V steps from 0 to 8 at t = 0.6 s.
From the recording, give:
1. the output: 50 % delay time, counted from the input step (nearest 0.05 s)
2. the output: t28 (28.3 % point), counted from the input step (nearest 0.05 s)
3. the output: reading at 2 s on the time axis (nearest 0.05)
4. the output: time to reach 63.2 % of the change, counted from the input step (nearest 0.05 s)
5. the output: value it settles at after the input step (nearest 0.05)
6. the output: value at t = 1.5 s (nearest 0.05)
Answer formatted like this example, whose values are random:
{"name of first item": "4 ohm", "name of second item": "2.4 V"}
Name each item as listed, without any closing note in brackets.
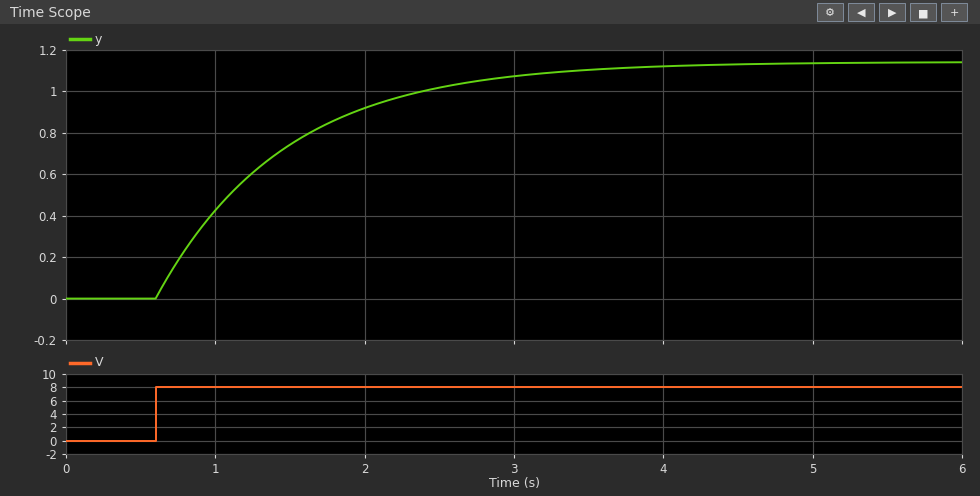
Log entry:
{"the output: 50 % delay time, counted from the input step": "0.60 s", "the output: t28 (28.3 % point), counted from the input step": "0.30 s", "the output: reading at 2 s on the time axis": "0.90", "the output: time to reach 63.2 % of the change, counted from the input step": "0.85 s", "the output: value it settles at after the input step": "1.15", "the output: value at t = 1.5 s": "0.75"}
